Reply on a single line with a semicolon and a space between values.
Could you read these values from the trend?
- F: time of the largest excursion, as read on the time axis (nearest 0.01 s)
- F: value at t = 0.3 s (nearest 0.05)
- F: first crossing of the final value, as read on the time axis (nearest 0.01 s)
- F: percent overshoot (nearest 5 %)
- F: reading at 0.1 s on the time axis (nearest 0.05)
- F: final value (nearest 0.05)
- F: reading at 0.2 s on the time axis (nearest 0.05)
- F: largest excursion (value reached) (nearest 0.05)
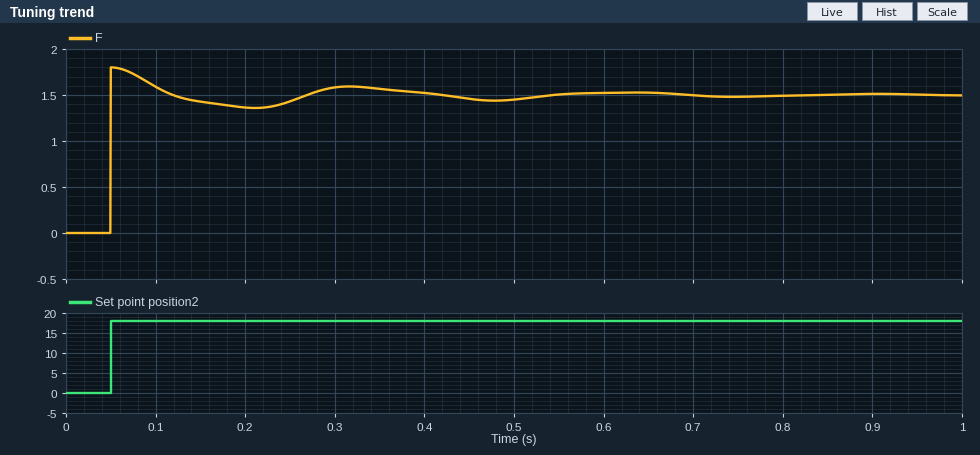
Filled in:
0.05 s; 1.60; 0.05 s; 20 %; 1.60; 1.50; 1.35; 1.80
